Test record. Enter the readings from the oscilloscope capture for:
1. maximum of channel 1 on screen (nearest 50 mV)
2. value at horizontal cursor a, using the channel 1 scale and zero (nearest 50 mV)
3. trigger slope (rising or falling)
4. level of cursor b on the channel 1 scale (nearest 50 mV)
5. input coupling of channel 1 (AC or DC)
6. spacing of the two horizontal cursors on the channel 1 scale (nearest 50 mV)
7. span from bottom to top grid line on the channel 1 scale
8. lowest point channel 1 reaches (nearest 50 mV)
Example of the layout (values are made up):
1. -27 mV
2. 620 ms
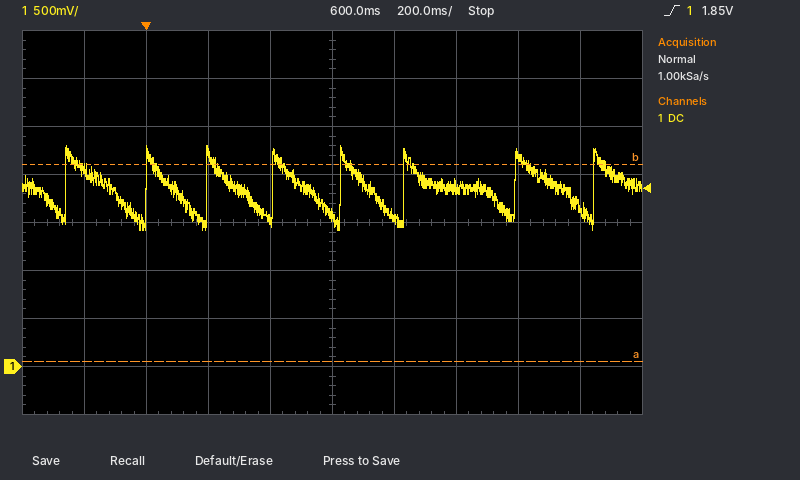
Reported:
1. 2.30 V
2. 50 mV
3. rising
4. 2.10 V
5. DC
6. 2.05 V
7. 4 V
8. 1.45 V
